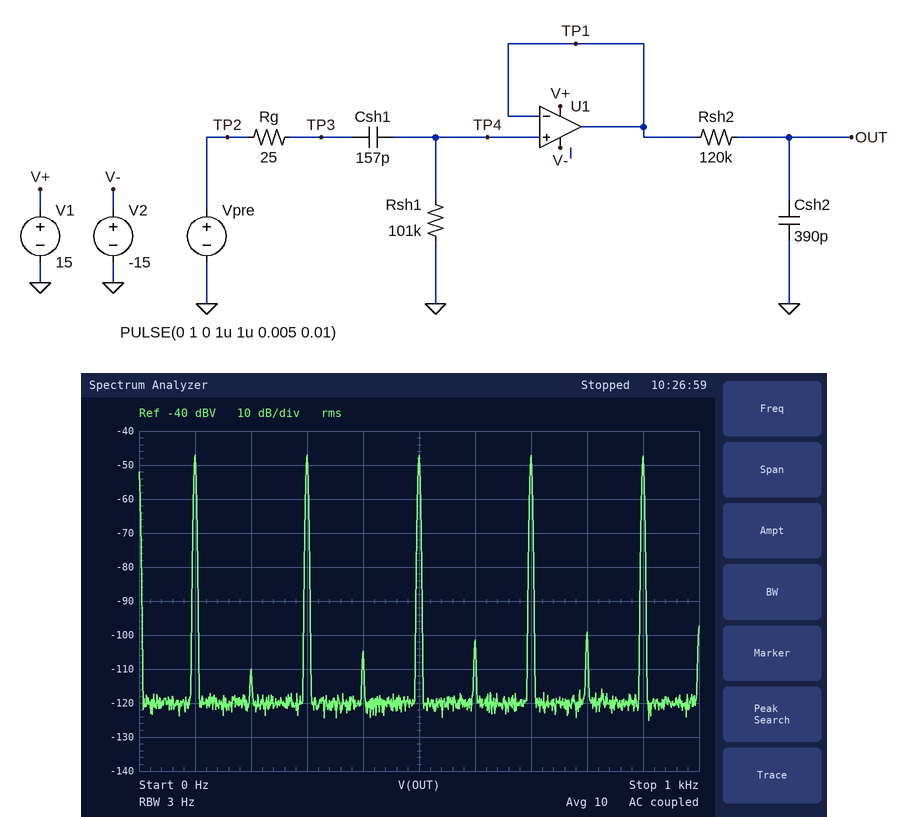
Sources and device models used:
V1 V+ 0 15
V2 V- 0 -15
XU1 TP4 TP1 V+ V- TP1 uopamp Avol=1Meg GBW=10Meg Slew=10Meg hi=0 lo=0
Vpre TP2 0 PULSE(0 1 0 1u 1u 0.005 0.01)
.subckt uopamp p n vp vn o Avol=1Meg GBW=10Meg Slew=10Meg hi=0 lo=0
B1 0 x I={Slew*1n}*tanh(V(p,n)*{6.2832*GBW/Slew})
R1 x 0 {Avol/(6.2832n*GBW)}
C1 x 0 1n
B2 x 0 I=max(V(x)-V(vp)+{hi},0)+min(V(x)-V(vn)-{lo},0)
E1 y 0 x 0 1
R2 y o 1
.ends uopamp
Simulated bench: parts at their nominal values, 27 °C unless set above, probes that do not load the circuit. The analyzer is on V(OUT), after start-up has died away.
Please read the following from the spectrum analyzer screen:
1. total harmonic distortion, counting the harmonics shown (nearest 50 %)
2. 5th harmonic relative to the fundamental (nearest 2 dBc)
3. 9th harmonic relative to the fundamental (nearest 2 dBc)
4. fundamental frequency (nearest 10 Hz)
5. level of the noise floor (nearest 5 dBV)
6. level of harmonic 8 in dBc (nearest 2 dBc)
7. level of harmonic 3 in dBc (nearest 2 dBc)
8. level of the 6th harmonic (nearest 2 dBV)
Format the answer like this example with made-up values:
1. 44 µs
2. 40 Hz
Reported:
1. 200 %
2. 0 dBc
3. 0 dBc
4. 100 Hz
5. -120 dBV
6. -52 dBc
7. 0 dBc
8. -102 dBV
